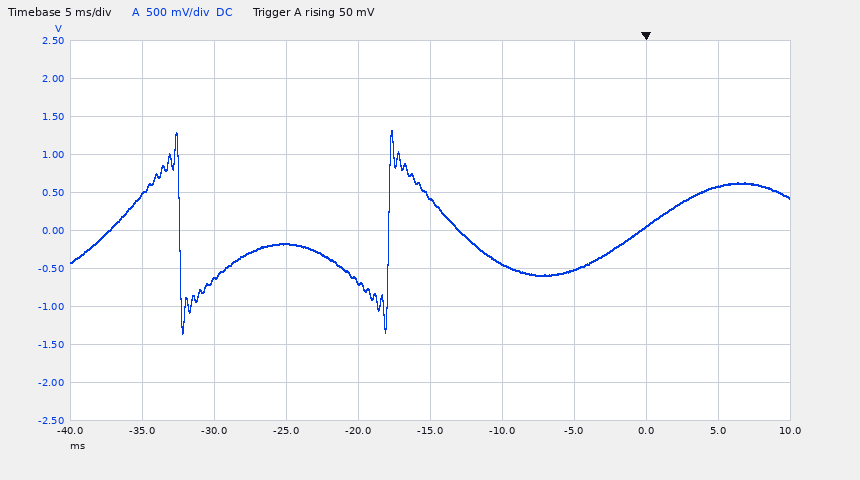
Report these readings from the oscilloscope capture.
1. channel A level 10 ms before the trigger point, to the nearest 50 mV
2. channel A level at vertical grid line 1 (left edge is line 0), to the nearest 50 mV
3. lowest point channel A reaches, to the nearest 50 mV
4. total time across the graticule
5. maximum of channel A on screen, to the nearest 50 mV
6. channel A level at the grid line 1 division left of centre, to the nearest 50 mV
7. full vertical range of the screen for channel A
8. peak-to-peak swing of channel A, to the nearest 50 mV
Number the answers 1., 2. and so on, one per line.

1. -450 mV
2. 450 mV
3. -1.35 V
4. 50 ms
5. 1.30 V
6. -650 mV
7. 5 V
8. 2.65 V
